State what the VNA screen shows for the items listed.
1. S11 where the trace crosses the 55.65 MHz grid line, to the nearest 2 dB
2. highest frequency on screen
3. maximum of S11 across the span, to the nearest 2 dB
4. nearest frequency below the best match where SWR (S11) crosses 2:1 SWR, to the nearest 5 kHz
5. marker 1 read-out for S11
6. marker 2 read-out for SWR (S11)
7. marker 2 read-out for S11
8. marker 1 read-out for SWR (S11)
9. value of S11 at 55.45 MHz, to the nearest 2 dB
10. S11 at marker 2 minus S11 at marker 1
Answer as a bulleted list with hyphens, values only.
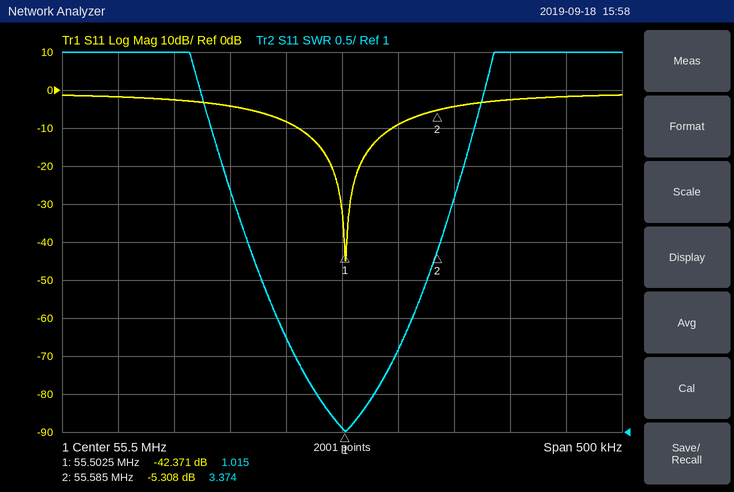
- -2 dB
- 55.75 MHz
- -2 dB
- 55.460 MHz
- -42.371 dB
- 3.374
- -5.308 dB
- 1.015
- -8 dB
- 37.063 dB
